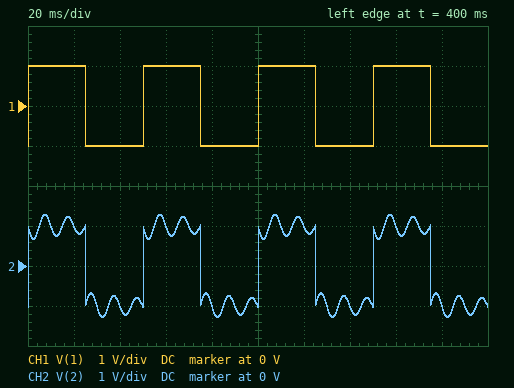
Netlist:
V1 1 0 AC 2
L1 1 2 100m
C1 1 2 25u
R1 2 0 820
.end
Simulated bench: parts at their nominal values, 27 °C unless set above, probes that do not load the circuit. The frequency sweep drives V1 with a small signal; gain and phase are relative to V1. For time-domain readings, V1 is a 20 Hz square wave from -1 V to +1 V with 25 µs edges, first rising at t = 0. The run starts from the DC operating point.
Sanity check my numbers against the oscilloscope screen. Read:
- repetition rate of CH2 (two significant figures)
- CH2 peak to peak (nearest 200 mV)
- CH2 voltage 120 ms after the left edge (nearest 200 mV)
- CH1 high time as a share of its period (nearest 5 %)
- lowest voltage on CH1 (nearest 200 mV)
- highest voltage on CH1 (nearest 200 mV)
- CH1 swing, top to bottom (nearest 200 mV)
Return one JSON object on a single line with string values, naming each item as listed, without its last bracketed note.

{"repetition rate of CH2": "20 Hz", "CH2 peak to peak": "2.6 V", "CH2 voltage 120 ms after the left edge": "1.0 V", "CH1 high time as a share of its period": "50 %", "lowest voltage on CH1": "-1.0 V", "highest voltage on CH1": "1.0 V", "CH1 swing, top to bottom": "2.0 V"}
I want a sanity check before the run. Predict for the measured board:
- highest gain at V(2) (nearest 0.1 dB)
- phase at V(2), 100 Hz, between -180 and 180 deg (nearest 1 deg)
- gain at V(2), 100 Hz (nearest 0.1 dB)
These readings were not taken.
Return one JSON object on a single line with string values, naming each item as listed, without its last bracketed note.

{"highest gain at V(2)": "0 dB", "phase at V(2), 100 Hz, between -180 and 180 deg": "-80 deg", "gain at V(2), 100 Hz": "-15.5 dB"}
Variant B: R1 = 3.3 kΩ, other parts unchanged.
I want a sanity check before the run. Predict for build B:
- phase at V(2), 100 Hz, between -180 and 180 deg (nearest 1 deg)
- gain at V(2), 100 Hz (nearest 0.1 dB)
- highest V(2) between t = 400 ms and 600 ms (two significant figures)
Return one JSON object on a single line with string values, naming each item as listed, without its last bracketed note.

{"phase at V(2), 100 Hz, between -180 and 180 deg": "-56 deg", "gain at V(2), 100 Hz": "-5.0 dB", "highest V(2) between t = 400 ms and 600 ms": "1.2 V"}
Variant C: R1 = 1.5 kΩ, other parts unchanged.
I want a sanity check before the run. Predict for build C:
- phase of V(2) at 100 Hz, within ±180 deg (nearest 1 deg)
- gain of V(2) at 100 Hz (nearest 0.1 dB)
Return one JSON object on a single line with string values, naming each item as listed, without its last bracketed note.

{"phase of V(2) at 100 Hz, within ±180 deg": "-73 deg", "gain of V(2) at 100 Hz": "-10.5 dB"}
